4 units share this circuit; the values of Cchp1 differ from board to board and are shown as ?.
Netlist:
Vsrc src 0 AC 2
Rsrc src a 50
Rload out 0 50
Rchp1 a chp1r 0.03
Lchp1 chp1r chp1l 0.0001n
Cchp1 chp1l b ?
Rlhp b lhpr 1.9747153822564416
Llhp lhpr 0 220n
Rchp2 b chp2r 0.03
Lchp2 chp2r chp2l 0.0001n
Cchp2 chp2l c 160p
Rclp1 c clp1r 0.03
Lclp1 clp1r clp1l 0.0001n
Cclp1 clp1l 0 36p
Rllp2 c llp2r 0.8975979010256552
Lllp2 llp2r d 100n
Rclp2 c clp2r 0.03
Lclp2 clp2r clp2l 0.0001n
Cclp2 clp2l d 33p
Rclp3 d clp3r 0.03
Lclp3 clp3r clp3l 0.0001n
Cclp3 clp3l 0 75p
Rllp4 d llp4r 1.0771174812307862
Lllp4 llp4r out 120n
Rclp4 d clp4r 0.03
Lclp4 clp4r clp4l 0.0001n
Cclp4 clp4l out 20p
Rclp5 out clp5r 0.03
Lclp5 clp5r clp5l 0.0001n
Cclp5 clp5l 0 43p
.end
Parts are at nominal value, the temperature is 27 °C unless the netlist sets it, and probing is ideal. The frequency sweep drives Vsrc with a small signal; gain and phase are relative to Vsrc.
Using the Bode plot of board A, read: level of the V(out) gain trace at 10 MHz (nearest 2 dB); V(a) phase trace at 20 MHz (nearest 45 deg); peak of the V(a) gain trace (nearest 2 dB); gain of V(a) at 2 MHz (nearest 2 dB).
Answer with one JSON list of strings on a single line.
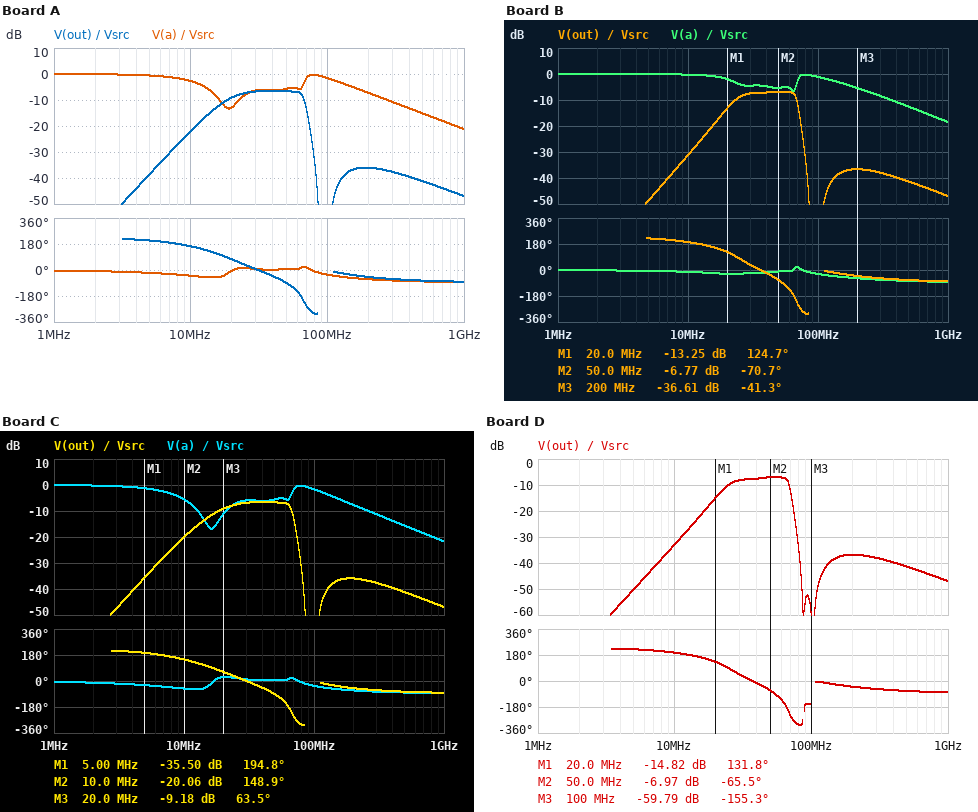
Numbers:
["-22 dB", "0 deg", "0 dB", "0 dB"]
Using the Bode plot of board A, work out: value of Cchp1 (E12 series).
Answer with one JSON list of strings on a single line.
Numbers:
["220 pF"]
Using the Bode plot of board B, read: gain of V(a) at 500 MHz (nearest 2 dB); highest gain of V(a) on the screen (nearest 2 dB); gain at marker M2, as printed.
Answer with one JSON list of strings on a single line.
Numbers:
["-12 dB", "0 dB", "-6.77 dB"]
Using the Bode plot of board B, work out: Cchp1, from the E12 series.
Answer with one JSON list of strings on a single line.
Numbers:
["68 pF"]
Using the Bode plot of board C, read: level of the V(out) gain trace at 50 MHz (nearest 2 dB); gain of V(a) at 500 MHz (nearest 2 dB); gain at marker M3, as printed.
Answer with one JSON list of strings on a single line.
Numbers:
["-6 dB", "-16 dB", "-9.18 dB"]
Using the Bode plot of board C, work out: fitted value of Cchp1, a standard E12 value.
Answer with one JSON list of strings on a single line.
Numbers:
["330 pF"]
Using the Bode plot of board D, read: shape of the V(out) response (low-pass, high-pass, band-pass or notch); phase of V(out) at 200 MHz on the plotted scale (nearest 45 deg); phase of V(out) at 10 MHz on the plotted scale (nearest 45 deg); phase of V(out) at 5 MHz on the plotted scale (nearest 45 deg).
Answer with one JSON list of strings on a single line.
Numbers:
["band-pass", "-45 deg", "180 deg", "225 deg"]
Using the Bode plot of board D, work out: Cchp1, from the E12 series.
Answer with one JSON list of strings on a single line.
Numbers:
["56 pF"]
